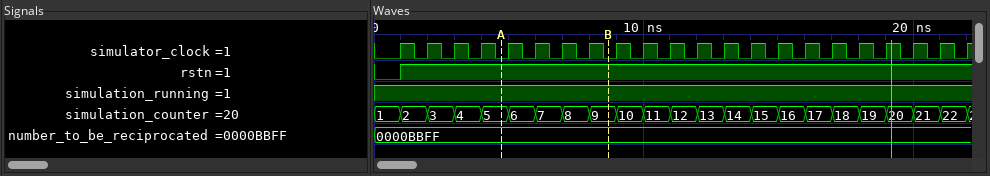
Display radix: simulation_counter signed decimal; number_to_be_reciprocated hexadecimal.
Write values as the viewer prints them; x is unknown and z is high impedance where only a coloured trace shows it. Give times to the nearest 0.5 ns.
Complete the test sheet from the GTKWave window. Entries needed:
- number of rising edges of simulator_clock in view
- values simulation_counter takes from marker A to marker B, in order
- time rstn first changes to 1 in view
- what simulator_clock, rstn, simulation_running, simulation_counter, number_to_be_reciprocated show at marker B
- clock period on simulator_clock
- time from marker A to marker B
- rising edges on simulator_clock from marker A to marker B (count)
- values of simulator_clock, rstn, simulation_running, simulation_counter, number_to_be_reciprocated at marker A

22
5, 6, 7, 8, 9
1 ns
simulator_clock=0, rstn=1, simulation_running=1, simulation_counter=9, number_to_be_reciprocated=0000BBFF
1 ns
4 ns
4
simulator_clock=0, rstn=1, simulation_running=1, simulation_counter=5, number_to_be_reciprocated=0000BBFF
